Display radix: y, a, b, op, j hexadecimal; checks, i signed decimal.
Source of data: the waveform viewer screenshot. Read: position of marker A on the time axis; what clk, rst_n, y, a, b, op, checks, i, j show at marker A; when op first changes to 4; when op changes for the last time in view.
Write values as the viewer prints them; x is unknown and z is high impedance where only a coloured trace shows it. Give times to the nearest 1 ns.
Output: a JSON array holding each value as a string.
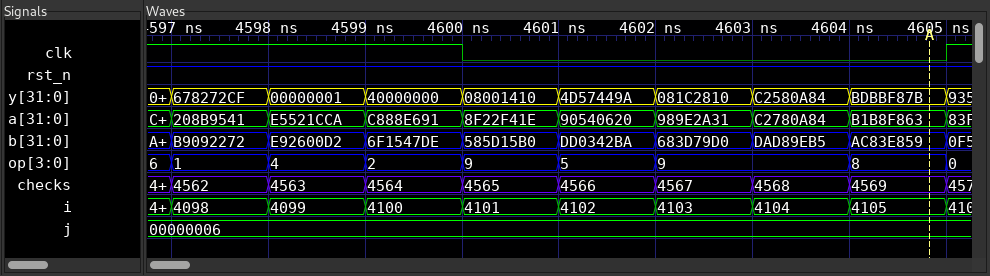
["4605 ns", "clk=0, rst_n=1, y=BDBBF87B, a=B1B8F863, b=AC83E859, op=8, checks=4569, i=4105, j=00000006", "4598 ns", "4605 ns"]
